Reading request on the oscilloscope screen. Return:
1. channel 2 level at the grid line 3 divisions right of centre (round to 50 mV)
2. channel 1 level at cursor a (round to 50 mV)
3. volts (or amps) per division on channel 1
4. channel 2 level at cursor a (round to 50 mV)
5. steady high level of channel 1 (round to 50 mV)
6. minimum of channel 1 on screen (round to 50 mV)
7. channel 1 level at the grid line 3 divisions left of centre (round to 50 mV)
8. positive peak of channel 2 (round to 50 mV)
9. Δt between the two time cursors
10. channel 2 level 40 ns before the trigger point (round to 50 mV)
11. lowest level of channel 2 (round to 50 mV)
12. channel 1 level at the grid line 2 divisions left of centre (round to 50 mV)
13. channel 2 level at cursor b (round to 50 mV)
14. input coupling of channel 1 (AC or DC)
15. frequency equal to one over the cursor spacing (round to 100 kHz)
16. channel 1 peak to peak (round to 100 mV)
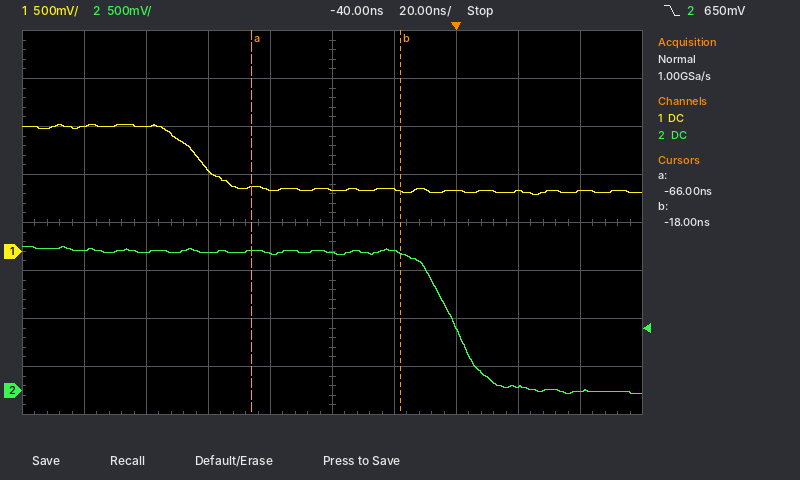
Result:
50 mV
650 mV
500 mV
1.45 V
1.30 V
600 mV
1.30 V
1.50 V
48 ns
1.45 V
-50 mV
850 mV
1.45 V
DC
20.8 MHz
700 mV
